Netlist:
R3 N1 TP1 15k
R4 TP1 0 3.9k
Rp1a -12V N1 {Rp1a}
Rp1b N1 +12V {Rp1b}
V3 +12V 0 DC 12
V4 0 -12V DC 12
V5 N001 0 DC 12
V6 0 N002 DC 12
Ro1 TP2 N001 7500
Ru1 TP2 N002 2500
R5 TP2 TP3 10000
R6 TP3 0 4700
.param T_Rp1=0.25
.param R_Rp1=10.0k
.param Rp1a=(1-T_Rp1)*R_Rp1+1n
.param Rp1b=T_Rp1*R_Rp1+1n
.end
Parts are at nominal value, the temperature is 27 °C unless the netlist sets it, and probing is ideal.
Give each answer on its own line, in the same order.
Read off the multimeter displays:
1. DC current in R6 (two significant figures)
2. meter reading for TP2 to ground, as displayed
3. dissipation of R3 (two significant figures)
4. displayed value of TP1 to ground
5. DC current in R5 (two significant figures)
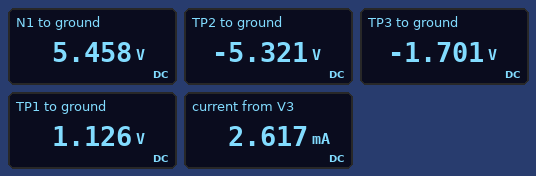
360 µA
-5.321 V
1.3 mW
1.126 V
360 µA
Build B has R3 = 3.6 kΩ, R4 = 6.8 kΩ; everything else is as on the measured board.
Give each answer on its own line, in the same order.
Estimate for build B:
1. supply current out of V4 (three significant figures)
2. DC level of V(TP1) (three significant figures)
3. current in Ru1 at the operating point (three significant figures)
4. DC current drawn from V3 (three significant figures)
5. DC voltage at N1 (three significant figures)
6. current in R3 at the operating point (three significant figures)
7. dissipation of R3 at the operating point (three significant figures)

2.28 mA
3.32 V
2.67 mA
2.77 mA
5.08 V
489 µA
860 µW
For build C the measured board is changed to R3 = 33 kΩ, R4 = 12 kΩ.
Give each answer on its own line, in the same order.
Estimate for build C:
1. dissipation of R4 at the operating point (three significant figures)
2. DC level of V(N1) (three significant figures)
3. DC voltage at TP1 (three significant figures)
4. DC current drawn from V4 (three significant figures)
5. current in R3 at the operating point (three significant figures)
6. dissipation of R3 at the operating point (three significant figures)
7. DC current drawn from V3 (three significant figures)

197 µW
5.76 V
1.54 V
2.37 mA
128 µA
541 µW
2.50 mA
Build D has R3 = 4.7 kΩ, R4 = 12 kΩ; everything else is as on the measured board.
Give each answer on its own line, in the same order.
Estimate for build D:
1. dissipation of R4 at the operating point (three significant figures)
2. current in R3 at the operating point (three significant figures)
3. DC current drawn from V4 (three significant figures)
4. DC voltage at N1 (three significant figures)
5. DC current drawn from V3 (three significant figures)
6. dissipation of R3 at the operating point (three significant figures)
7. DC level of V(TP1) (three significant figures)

1.25 mW
323 µA
2.32 mA
5.39 V
2.64 mA
490 µW
3.88 V
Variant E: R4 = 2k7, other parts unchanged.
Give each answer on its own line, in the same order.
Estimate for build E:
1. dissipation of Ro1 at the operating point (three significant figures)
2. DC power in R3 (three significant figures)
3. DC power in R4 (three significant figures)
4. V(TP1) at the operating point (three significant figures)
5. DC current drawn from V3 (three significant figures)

40.0 mW
1.41 mW
254 µW
828 mV
2.63 mA
